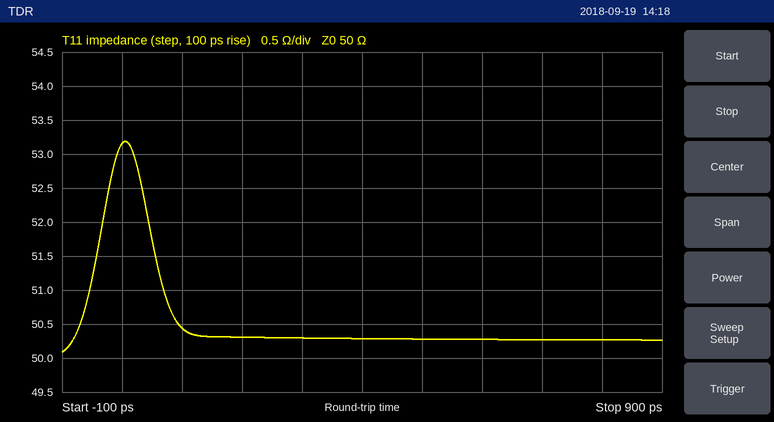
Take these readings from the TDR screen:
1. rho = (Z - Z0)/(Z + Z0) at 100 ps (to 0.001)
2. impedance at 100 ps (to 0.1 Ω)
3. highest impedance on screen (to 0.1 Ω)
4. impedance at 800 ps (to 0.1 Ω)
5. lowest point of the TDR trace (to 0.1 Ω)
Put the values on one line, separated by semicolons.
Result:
+0.004; 50.4 Ω; 53.2 Ω; 50.3 Ω; 50.1 Ω
